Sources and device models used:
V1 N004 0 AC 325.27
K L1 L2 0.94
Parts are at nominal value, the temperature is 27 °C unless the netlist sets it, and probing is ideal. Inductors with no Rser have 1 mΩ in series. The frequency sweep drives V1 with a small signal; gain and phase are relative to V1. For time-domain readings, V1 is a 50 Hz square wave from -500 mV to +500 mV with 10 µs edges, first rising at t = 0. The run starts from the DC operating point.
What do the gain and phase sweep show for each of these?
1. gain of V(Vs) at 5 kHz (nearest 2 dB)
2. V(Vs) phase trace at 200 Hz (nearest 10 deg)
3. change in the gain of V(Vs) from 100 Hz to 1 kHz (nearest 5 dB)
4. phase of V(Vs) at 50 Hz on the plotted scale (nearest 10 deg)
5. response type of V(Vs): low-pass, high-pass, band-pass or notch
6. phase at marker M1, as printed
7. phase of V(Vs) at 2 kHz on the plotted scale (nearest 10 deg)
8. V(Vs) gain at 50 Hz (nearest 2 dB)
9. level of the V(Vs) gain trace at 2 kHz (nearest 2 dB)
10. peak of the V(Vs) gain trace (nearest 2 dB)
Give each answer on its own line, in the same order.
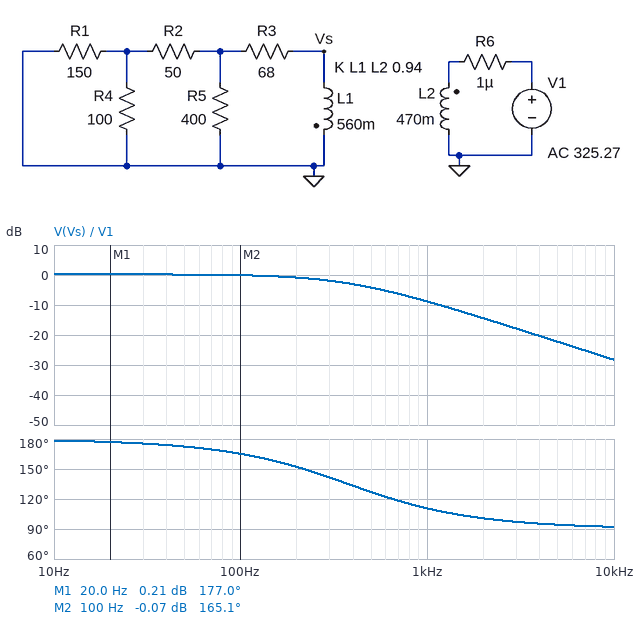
-22 dB
150 deg
-10 dB
170 deg
low-pass
177.0 deg
100 deg
0 dB
-14 dB
0 dB
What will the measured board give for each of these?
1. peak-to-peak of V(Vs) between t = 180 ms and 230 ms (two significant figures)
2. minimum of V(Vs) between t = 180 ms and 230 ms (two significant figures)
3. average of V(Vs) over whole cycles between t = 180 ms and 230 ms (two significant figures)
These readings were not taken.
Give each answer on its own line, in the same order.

1.0 V
-1.0 V
-510 mV
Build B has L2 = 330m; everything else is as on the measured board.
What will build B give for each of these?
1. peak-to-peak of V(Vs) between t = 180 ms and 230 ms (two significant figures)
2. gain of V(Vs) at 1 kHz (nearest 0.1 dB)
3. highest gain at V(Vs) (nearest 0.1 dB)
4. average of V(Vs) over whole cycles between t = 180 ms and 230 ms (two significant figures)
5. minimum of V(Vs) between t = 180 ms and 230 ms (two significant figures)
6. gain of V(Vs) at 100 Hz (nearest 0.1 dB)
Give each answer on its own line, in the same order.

1.2 V
-7.3 dB
1.8 dB
-610 mV
-1.2 V
1.5 dB
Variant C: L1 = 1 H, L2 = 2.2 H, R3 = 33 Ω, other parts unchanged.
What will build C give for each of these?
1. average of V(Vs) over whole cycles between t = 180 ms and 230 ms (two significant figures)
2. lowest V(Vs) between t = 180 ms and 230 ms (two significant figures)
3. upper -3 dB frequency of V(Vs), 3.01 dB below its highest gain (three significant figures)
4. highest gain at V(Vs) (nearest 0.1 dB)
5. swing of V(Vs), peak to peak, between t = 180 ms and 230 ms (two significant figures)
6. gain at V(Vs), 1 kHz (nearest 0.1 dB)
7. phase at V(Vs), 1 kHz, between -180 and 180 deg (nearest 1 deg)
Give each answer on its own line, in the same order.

-320 mV
-630 mV
163 Hz
-4.0 dB
630 mV
-19.8 dB
99 deg
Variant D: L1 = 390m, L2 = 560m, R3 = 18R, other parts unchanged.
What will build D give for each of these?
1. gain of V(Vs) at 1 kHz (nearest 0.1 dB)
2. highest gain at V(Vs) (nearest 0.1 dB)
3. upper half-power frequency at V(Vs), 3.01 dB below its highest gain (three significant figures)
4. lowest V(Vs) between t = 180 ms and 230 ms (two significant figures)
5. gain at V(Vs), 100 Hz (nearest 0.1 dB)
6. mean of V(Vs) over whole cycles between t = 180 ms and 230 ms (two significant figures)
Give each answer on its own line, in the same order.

-11.4 dB
-2.1 dB
366 Hz
-780 mV
-2.4 dB
-390 mV
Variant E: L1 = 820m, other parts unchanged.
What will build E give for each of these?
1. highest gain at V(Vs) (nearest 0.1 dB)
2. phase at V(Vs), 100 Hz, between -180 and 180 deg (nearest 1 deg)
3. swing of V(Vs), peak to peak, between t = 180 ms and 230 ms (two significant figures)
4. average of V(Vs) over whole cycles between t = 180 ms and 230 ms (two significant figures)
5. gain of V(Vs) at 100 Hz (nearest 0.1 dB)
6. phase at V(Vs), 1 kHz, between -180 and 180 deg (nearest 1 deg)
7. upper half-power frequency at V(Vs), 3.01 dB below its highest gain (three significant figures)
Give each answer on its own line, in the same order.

1.9 dB
159 deg
1.2 V
-620 mV
1.3 dB
104 deg
257 Hz
